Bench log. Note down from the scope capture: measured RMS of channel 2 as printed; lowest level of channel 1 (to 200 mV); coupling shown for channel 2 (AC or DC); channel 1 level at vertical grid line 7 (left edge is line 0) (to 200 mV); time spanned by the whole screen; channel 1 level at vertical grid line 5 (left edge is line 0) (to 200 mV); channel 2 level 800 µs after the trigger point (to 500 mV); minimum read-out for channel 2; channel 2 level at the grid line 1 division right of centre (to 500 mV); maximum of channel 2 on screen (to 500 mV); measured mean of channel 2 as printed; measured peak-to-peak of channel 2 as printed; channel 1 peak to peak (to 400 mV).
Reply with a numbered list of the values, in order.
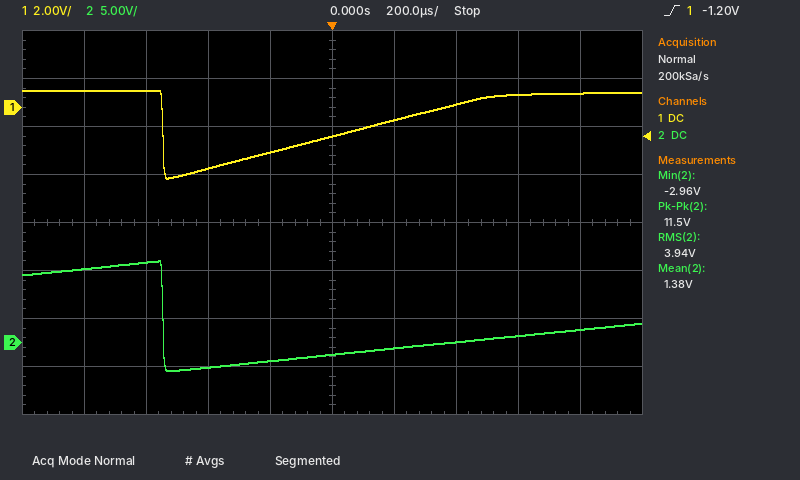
1. 3.94 V
2. -3.0 V
3. DC
4. 200 mV
5. 2 ms
6. -1.2 V
7. 1.5 V
8. -2.96 V
9. -500 mV
10. 8.5 V
11. 1.38 V
12. 11.5 V
13. 3.6 V
